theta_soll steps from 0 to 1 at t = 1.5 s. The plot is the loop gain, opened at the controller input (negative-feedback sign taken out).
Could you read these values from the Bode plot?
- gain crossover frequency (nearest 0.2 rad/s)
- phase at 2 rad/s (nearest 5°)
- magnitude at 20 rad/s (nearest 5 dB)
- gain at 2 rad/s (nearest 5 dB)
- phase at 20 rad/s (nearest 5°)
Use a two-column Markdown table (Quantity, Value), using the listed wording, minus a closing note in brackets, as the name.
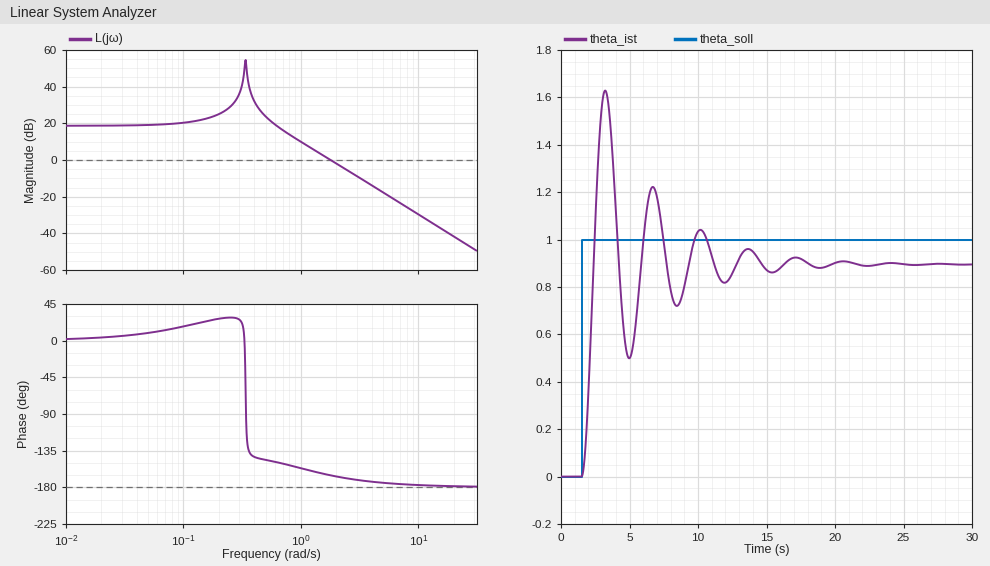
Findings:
| Quantity | Value |
|---|---|
| gain crossover frequency | 1.8 rad/s |
| phase at 2 rad/s | -165° |
| magnitude at 20 rad/s | -40 dB |
| gain at 2 rad/s | 0 dB |
| phase at 20 rad/s | -180° |
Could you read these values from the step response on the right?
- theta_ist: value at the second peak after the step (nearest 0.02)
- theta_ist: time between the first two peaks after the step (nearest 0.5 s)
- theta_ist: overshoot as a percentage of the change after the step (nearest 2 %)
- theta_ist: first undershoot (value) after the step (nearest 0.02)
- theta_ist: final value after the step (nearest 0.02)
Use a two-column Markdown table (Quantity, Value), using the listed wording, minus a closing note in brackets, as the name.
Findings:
| Quantity | Value |
|---|---|
| theta_ist: value at the second peak after the step | 1.22 |
| theta_ist: time between the first two peaks after the step | 3.5 s |
| theta_ist: overshoot as a percentage of the change after the step | 82 % |
| theta_ist: first undershoot (value) after the step | 0.50 |
| theta_ist: final value after the step | 0.90 |
